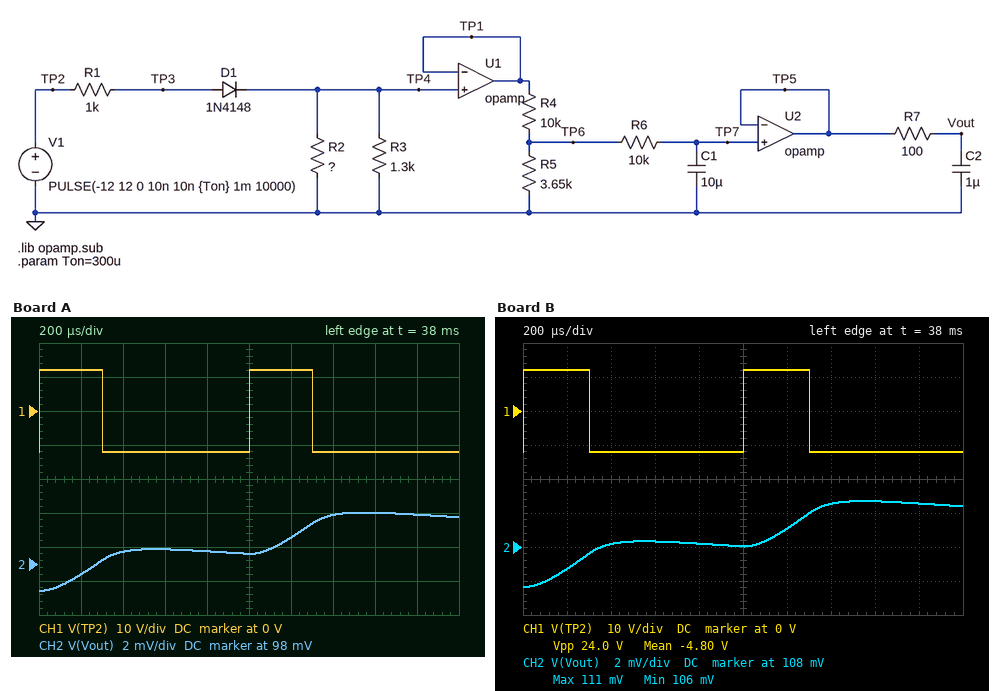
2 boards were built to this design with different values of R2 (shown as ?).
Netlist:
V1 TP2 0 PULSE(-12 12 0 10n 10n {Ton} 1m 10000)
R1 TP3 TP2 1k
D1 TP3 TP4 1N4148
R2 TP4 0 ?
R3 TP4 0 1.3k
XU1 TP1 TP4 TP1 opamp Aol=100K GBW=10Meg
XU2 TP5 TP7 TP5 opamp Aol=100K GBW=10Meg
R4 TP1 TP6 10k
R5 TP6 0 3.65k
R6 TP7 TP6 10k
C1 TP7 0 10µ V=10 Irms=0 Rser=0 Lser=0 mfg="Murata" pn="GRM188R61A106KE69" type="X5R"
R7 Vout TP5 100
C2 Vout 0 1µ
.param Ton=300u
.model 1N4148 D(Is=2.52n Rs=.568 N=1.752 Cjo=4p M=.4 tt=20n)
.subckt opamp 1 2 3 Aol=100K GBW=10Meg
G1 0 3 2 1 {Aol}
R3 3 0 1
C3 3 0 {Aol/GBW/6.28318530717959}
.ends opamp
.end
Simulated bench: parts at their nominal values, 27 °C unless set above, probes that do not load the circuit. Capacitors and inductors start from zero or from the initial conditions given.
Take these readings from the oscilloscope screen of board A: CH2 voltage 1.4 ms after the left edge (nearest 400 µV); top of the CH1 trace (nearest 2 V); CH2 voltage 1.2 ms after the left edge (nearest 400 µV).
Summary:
100.8 mV
12 V
99.6 mV
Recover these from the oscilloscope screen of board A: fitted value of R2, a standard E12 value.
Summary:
1.5 kΩ
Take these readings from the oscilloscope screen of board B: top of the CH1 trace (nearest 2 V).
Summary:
12 V
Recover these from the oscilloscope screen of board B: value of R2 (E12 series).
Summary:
2.2 kΩ
